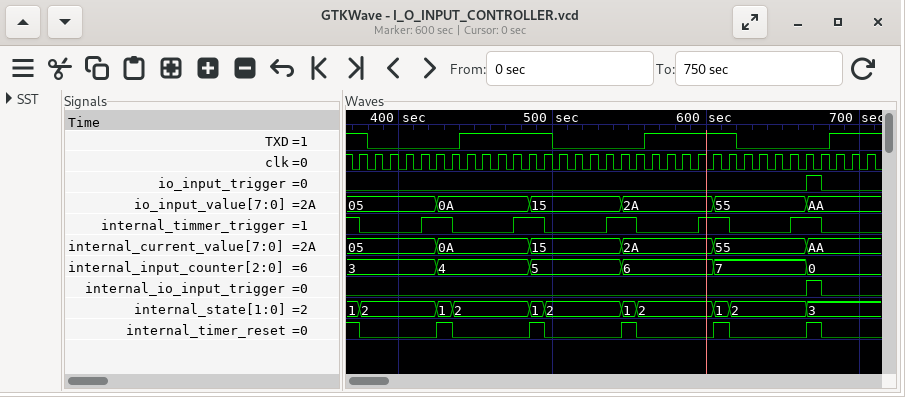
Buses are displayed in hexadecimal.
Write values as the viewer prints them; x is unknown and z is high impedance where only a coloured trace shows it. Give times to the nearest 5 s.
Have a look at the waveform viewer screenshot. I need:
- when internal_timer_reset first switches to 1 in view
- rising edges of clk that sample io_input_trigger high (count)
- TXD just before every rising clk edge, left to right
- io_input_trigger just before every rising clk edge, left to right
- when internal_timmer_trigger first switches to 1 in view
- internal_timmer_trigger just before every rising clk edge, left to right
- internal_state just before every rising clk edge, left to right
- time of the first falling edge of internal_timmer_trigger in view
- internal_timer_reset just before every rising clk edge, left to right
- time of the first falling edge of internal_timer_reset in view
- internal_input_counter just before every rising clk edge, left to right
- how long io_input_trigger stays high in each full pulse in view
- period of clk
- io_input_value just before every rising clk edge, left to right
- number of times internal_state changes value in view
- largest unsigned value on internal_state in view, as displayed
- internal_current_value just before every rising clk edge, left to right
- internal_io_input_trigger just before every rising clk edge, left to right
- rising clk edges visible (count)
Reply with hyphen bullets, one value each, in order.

- 425 s
- 1
- 1 0 0 0 0 0 0 1 1 1 1 1 1 0 0 0 0 0 0 1 1 1 1 1 1 0 0 0 0 0 0 1 1 1
- 0 0 0 0 0 0 0 0 0 0 0 0 0 0 0 0 0 0 0 0 0 0 0 0 0 0 0 0 0 0 1 0 0 0
- 415 s
- 1 0 0 0 0 1 1 0 0 0 0 1 1 0 0 0 0 1 1 0 0 0 0 1 1 0 0 0 0 1 1 0 0 0
- 1, 2, 2, 2, 2, 2, 1, 2, 2, 2, 2, 2, 1, 2, 2, 2, 2, 2, 1, 2, 2, 2, 2, 2, 1, 2, 2, 2, 2, 2, 3, 3, 3, 3
- 375 s
- 1 0 0 0 0 0 1 0 0 0 0 0 1 0 0 0 0 0 1 0 0 0 0 0 1 0 0 0 0 0 1 0 0 0
- 375 s
- 3, 3, 3, 3, 3, 3, 4, 4, 4, 4, 4, 4, 5, 5, 5, 5, 5, 5, 6, 6, 6, 6, 6, 6, 7, 7, 7, 7, 7, 7, 0, 0, 0, 0
- 10 s
- 10 s
- 05, 05, 05, 05, 05, 05, 0A, 0A, 0A, 0A, 0A, 0A, 15, 15, 15, 15, 15, 15, 2A, 2A, 2A, 2A, 2A, 2A, 55, 55, 55, 55, 55, 55, AA, AA, AA, AA
- 10
- 3
- 05, 05, 05, 05, 05, 05, 0A, 0A, 0A, 0A, 0A, 0A, 15, 15, 15, 15, 15, 15, 2A, 2A, 2A, 2A, 2A, 2A, 55, 55, 55, 55, 55, 55, AA, AA, AA, AA
- 0 0 0 0 0 0 0 0 0 0 0 0 0 0 0 0 0 0 0 0 0 0 0 0 0 0 0 0 0 0 1 0 0 0
- 34
